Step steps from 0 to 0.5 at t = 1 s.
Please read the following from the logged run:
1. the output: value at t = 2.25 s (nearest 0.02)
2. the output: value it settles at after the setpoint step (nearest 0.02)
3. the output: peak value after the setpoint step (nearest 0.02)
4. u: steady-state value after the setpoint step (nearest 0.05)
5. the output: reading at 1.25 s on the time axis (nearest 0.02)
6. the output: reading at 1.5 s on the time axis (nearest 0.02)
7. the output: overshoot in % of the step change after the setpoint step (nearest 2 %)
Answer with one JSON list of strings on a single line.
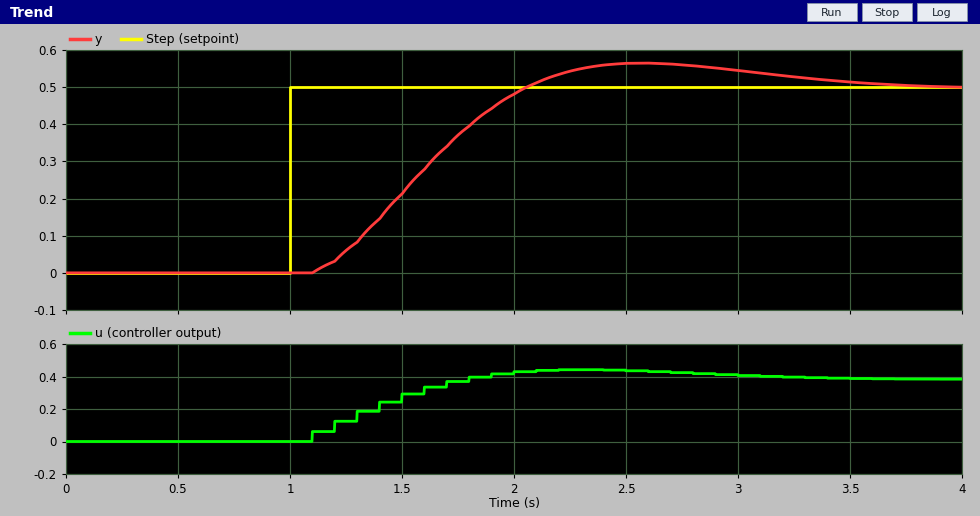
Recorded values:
["0.54", "0.50", "0.56", "0.40", "0.06", "0.22", "12 %"]
